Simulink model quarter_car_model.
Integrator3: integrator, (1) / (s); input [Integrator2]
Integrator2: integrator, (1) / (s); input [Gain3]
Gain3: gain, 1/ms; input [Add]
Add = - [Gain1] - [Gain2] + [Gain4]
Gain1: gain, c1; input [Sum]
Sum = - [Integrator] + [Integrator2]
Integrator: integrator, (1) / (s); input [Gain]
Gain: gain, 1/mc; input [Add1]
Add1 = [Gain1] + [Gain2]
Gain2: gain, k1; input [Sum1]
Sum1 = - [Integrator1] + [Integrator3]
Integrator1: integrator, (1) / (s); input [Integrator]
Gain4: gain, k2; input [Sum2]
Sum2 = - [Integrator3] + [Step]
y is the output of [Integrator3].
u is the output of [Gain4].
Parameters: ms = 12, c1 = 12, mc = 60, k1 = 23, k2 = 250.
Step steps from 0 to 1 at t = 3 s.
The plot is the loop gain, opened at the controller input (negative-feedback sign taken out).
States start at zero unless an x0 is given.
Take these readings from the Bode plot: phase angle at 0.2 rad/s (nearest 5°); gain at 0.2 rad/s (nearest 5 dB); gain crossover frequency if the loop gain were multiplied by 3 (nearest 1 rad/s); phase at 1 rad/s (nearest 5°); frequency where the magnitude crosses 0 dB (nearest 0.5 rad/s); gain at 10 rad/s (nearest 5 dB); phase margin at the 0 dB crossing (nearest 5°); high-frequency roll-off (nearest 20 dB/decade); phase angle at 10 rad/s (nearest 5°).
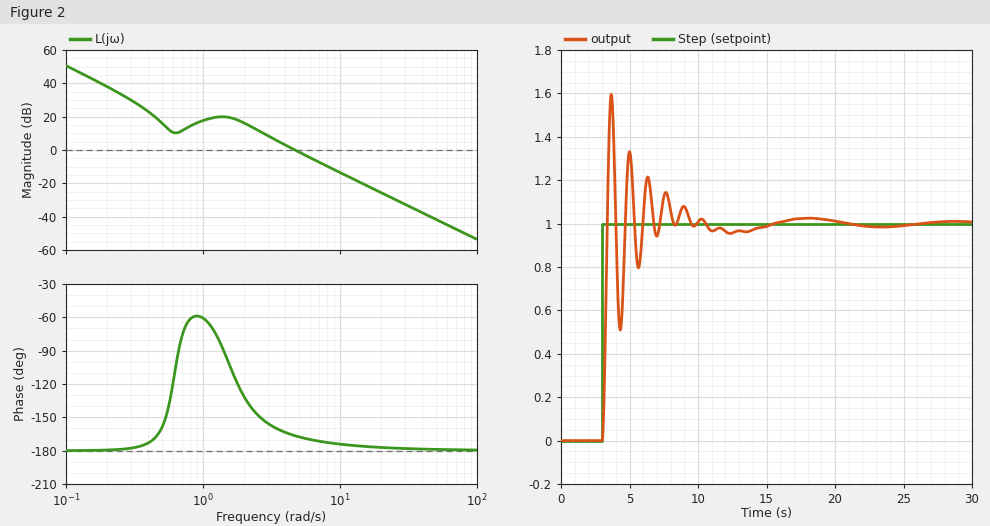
-180°
40 dB
8 rad/s
-60°
4.5 rad/s
-15 dB
15°
-40 dB/decade
-175°
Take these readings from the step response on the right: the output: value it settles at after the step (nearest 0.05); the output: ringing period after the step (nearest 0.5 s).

1.00
1.5 s
